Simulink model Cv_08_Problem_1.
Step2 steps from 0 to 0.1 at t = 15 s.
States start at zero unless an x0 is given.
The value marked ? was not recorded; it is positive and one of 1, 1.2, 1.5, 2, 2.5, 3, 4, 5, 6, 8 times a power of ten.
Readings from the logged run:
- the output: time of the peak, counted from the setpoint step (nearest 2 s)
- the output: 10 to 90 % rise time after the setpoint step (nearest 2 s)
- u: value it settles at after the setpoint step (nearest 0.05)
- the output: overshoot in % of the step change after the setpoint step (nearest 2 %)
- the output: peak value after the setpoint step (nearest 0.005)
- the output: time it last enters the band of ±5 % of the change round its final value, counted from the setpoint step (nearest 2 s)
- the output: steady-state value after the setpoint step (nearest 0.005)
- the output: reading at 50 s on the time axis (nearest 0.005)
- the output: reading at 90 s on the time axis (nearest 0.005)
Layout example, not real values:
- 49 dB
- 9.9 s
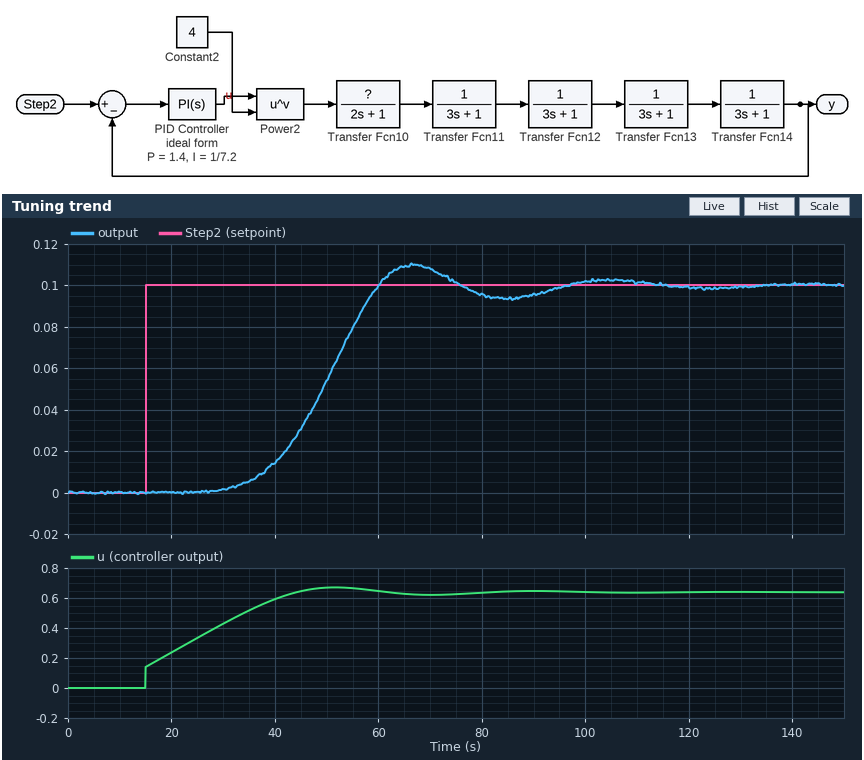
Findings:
- 52 s
- 20 s
- 0.65
- 10 %
- 0.110
- 74 s
- 0.100
- 0.055
- 0.095
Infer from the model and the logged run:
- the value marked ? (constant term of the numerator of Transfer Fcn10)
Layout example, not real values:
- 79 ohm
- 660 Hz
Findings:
- 0.6
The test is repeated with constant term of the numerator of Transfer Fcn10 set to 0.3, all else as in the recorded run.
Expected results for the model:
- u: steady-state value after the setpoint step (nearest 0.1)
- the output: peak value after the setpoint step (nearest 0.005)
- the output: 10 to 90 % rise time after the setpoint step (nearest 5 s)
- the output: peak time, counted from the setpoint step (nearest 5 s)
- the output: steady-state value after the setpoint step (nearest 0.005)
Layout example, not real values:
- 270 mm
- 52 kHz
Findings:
- 0.8
- 0.105
- 25 s
- 60 s
- 0.100
